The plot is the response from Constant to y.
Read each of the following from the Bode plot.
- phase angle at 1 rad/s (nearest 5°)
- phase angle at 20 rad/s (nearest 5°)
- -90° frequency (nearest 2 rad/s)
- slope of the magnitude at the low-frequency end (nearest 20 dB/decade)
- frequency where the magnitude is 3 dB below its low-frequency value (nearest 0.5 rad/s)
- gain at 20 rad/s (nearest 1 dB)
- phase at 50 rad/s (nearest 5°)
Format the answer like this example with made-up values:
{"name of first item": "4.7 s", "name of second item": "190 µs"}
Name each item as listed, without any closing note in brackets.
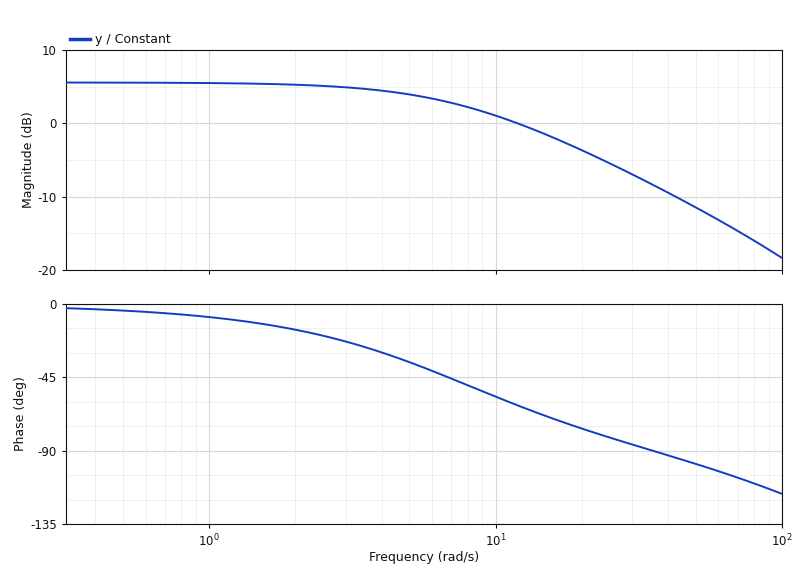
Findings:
{"phase angle at 1 rad/s": "-10°", "phase angle at 20 rad/s": "-75°", "-90° frequency": "36 rad/s", "slope of the magnitude at the low-frequency end": "0 dB/decade", "frequency where the magnitude is 3 dB below its low-frequency value": "7.5 rad/s", "gain at 20 rad/s": "-4 dB", "phase at 50 rad/s": "-100°"}
